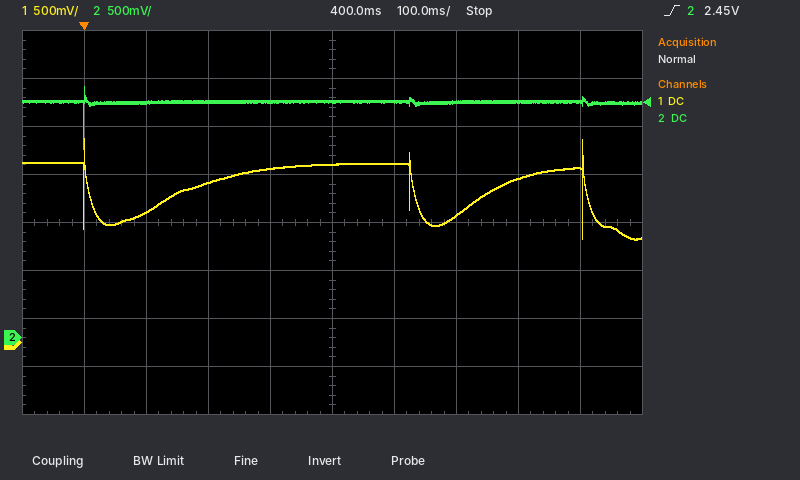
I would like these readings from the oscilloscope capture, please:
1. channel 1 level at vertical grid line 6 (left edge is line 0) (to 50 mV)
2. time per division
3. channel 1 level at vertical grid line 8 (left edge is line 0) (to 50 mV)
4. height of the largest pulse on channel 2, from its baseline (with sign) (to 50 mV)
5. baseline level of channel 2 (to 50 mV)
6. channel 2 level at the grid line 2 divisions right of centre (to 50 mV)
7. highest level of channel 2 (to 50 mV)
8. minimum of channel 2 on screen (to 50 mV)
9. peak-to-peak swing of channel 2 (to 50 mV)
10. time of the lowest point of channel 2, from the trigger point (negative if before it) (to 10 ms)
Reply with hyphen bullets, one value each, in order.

- 1.85 V
- 100 ms
- 1.70 V
- -500 mV
- 2.45 V
- 2.45 V
- 2.60 V
- 1.95 V
- 650 mV
- 0 ms
